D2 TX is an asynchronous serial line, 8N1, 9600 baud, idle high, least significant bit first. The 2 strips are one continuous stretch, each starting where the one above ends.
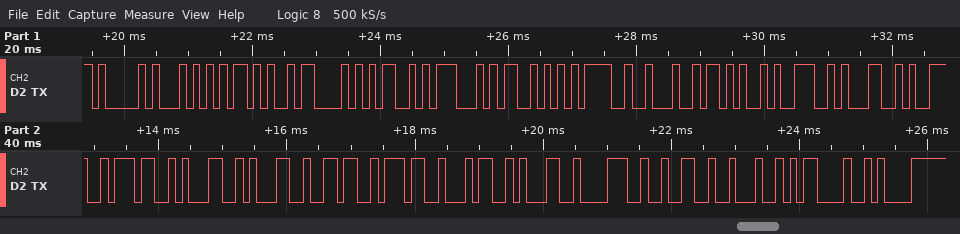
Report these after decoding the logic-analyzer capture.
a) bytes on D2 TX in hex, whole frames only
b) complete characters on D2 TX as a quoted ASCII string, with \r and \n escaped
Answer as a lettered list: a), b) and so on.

a) 41 54 2B 43 4D 47 53 3D 22 2B 39 31 39 37 31 31 36 37 34 31 38 32 22 0D 0A
b) "AT+CMGS=\"+919711674182\"\r\n"
